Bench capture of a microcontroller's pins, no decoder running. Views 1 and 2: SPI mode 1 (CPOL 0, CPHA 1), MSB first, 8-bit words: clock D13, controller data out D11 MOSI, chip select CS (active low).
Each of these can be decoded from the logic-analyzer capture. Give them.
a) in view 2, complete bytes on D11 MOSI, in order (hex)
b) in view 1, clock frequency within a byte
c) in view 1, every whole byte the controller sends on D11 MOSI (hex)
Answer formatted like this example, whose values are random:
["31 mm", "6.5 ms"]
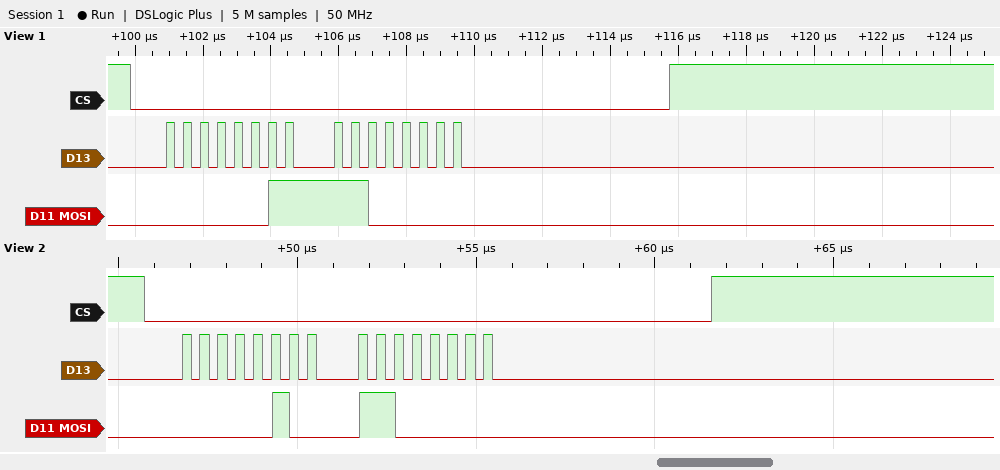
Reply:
["0x04 0xC0", "2 MHz", "03 C0"]
